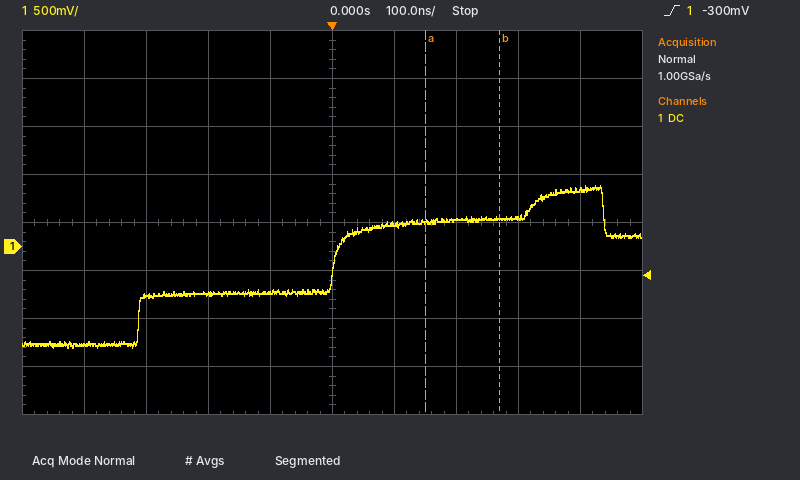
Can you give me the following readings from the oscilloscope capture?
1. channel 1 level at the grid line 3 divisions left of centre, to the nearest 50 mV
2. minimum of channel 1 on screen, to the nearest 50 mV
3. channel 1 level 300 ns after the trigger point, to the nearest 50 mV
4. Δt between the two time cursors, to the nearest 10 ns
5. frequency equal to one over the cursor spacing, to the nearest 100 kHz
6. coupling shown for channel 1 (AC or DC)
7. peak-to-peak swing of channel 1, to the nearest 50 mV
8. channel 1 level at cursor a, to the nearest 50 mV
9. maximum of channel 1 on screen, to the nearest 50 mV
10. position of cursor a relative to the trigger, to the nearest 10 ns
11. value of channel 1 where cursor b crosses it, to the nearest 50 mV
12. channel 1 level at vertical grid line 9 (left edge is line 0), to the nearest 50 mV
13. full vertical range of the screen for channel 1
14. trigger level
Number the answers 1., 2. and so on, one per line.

1. -500 mV
2. -1.05 V
3. 300 mV
4. 120 ns
5. 8.3 MHz
6. DC
7. 1.70 V
8. 250 mV
9. 650 mV
10. +150 ns
11. 300 mV
12. 600 mV
13. 4 V
14. -300 mV
